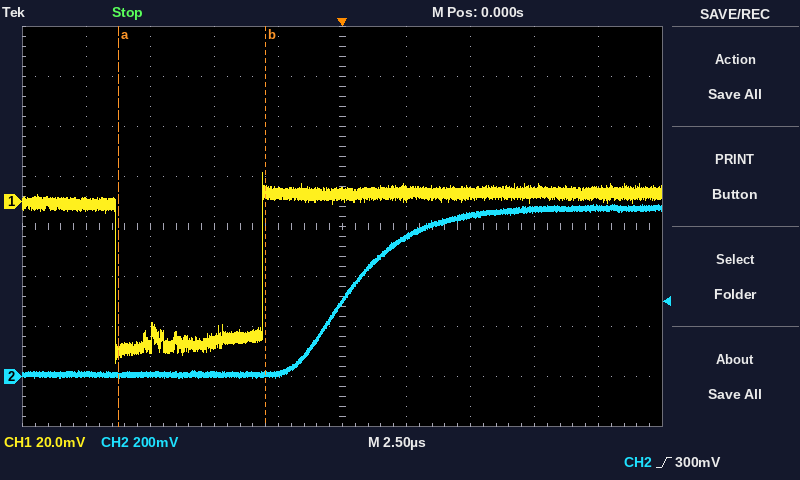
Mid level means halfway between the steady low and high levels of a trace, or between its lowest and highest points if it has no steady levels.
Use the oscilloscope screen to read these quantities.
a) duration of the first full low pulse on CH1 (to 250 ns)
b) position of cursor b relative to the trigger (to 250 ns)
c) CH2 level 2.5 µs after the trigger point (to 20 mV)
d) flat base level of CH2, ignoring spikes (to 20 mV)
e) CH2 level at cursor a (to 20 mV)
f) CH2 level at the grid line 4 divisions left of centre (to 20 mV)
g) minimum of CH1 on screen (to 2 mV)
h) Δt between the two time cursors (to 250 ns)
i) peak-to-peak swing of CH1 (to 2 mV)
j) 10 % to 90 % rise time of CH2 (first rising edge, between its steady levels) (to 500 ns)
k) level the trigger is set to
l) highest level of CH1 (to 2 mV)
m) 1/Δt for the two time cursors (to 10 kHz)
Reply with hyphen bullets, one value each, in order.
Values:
- 5.75 µs
- -3.00 µs
- 560 mV
- 0 mV
- 0 mV
- 0 mV
- -64 mV
- 5.75 µs
- 76 mV
- 5.0 µs
- 300 mV
- 12 mV
- 170 kHz
